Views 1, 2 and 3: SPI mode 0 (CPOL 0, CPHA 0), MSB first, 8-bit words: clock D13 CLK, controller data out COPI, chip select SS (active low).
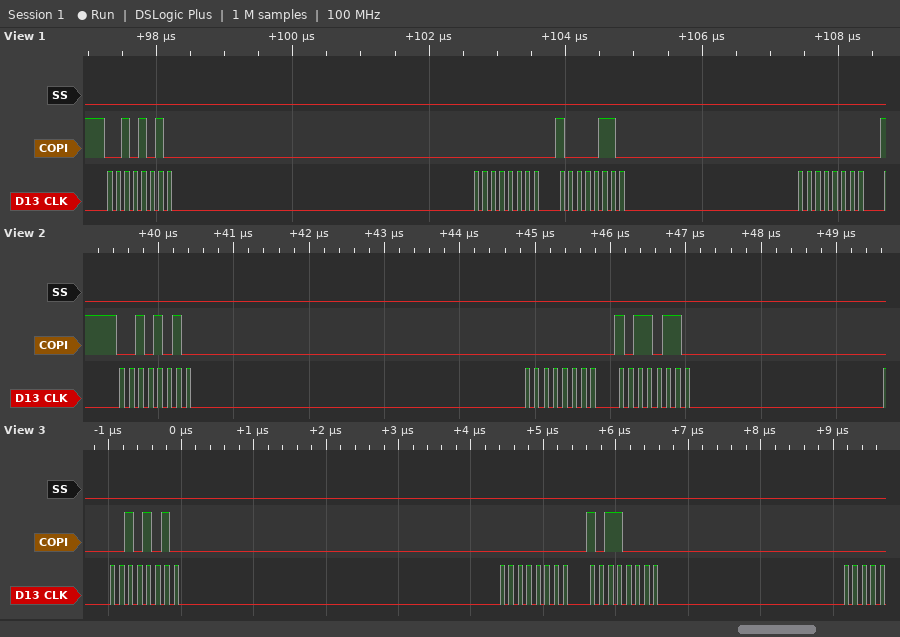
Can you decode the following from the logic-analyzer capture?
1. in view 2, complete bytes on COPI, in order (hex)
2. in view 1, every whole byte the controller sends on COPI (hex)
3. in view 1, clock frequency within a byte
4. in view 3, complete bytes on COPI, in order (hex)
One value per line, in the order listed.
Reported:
2A 00 B6
0x2A 0x00 0x86 0x00
8 MHz
0x2A 0x00 0xB0
